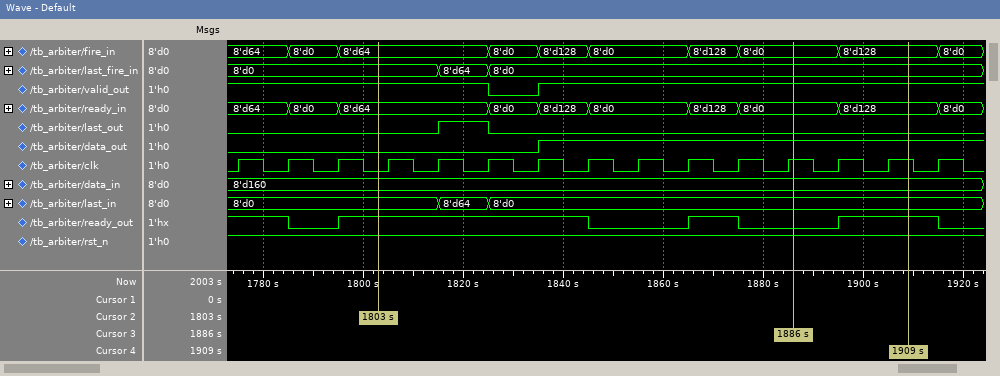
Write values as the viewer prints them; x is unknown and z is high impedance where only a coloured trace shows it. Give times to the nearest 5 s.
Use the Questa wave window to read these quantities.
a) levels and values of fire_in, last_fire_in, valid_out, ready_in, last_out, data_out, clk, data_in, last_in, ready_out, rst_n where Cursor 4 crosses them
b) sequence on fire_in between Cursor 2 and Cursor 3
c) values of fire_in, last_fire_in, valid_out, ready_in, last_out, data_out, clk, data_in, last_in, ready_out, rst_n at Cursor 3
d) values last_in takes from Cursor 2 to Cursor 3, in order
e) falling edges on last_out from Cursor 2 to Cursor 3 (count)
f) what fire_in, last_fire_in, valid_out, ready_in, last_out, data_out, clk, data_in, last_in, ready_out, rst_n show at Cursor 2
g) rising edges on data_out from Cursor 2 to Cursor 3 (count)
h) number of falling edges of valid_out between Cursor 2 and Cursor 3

fire_in=8'd128, last_fire_in=8'd0, valid_out=1, ready_in=8'd128, last_out=0, data_out=1, clk=1, data_in=8'd160, last_in=8'd0, ready_out=1, rst_n=1
8'd64, 8'd0, 8'd128, 8'd0, 8'd128, 8'd0
fire_in=8'd0, last_fire_in=8'd0, valid_out=1, ready_in=8'd0, last_out=0, data_out=1, clk=1, data_in=8'd160, last_in=8'd0, ready_out=0, rst_n=1
8'd0, 8'd64, 8'd0
1
fire_in=8'd64, last_fire_in=8'd0, valid_out=1, ready_in=8'd64, last_out=0, data_out=0, clk=0, data_in=8'd160, last_in=8'd0, ready_out=1, rst_n=1
1
1
